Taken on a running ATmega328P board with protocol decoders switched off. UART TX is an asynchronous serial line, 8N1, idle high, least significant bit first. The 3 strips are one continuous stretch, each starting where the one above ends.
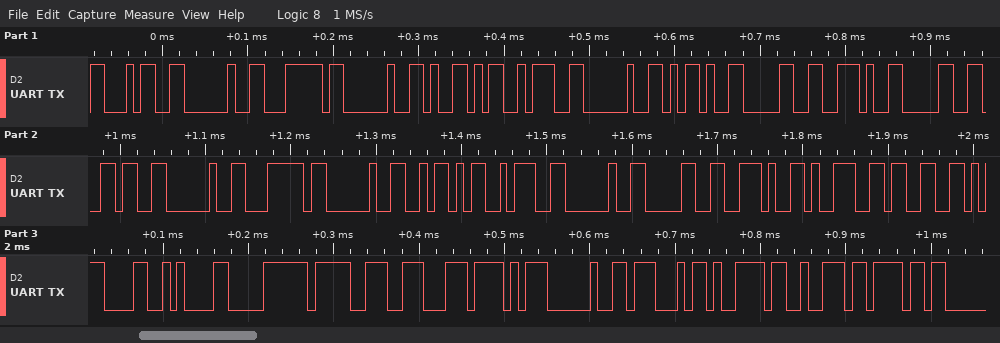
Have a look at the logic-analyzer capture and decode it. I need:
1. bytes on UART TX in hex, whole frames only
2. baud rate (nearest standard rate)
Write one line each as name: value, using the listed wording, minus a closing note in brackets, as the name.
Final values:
bytes on UART TX in hex, whole frames only: 0x34 0x20 0x7C 0x20 0x59 0x3A 0x20 0x2D 0x30 0x2E 0x30 0x36 0x20 0x7C 0x20 0x5A 0x3A 0x20 0x30 0x2E 0x39 0x33 0x0D 0x0A 0xF0 0x9F 0x8E 0xAF 0x20 0x47 0x79 0x72 0x6F
baud rate: 115200 baud
